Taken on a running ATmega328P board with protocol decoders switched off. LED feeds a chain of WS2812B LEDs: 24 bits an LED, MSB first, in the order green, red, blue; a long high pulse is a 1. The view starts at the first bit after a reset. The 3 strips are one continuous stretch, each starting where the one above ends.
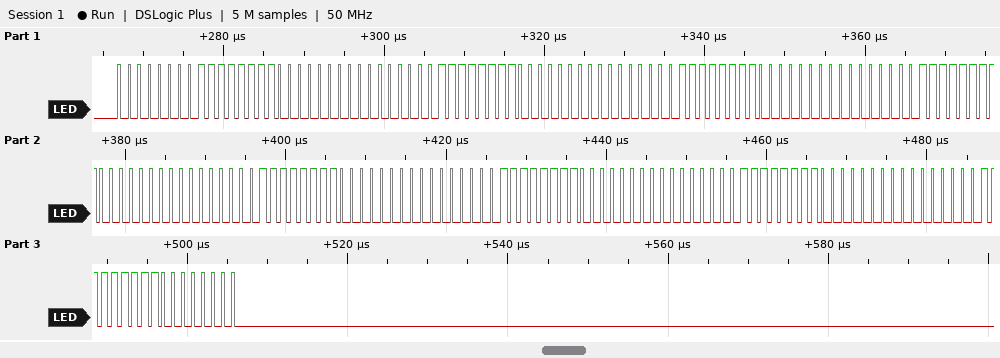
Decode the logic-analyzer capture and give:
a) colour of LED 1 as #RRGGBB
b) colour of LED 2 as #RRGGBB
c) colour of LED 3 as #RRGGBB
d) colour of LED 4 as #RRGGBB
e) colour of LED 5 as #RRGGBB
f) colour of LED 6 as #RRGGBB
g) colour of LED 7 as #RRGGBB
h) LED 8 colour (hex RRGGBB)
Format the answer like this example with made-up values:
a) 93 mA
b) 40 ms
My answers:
a) #FF0000
b) #FF0000
c) #FF0000
d) #FF0000
e) #FF0000
f) #FF0000
g) #FF0000
h) #FF0000
